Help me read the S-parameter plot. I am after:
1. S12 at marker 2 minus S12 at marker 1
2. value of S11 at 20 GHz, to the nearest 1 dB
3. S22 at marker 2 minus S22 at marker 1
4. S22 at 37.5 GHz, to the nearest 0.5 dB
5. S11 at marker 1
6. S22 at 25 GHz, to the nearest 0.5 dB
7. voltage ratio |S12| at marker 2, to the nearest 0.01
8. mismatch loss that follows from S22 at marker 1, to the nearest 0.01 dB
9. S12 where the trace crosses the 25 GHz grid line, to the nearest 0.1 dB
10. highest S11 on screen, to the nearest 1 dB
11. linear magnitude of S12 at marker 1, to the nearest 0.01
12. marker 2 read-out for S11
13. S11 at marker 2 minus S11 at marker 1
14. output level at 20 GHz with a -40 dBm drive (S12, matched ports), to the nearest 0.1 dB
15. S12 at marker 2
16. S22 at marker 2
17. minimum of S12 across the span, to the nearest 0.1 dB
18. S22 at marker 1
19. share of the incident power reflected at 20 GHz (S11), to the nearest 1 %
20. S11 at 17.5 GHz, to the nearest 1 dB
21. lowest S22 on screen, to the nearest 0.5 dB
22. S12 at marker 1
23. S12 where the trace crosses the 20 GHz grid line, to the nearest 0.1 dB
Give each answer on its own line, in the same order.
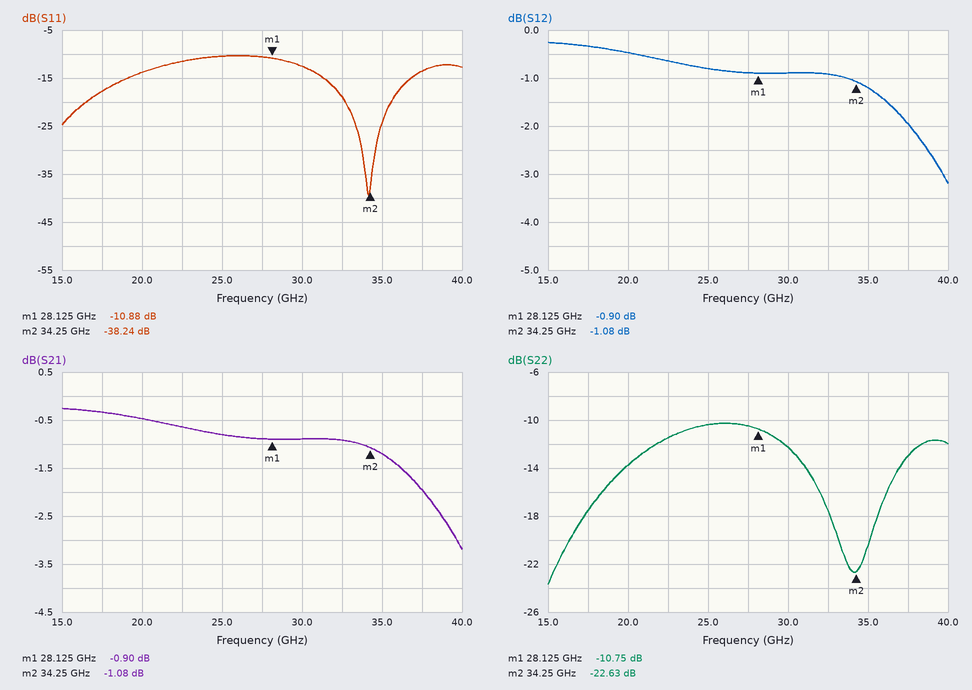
-0.18 dB
-14 dB
-11.88 dB
-13.0 dB
-10.88 dB
-10.5 dB
0.88
0.38 dB
-0.8 dB
-10 dB
0.90
-38.24 dB
-27.36 dB
-40.5 dBm
-1.08 dB
-22.63 dB
-3.2 dB
-10.75 dB
4 %
-18 dB
-23.5 dB
-0.90 dB
-0.5 dB
